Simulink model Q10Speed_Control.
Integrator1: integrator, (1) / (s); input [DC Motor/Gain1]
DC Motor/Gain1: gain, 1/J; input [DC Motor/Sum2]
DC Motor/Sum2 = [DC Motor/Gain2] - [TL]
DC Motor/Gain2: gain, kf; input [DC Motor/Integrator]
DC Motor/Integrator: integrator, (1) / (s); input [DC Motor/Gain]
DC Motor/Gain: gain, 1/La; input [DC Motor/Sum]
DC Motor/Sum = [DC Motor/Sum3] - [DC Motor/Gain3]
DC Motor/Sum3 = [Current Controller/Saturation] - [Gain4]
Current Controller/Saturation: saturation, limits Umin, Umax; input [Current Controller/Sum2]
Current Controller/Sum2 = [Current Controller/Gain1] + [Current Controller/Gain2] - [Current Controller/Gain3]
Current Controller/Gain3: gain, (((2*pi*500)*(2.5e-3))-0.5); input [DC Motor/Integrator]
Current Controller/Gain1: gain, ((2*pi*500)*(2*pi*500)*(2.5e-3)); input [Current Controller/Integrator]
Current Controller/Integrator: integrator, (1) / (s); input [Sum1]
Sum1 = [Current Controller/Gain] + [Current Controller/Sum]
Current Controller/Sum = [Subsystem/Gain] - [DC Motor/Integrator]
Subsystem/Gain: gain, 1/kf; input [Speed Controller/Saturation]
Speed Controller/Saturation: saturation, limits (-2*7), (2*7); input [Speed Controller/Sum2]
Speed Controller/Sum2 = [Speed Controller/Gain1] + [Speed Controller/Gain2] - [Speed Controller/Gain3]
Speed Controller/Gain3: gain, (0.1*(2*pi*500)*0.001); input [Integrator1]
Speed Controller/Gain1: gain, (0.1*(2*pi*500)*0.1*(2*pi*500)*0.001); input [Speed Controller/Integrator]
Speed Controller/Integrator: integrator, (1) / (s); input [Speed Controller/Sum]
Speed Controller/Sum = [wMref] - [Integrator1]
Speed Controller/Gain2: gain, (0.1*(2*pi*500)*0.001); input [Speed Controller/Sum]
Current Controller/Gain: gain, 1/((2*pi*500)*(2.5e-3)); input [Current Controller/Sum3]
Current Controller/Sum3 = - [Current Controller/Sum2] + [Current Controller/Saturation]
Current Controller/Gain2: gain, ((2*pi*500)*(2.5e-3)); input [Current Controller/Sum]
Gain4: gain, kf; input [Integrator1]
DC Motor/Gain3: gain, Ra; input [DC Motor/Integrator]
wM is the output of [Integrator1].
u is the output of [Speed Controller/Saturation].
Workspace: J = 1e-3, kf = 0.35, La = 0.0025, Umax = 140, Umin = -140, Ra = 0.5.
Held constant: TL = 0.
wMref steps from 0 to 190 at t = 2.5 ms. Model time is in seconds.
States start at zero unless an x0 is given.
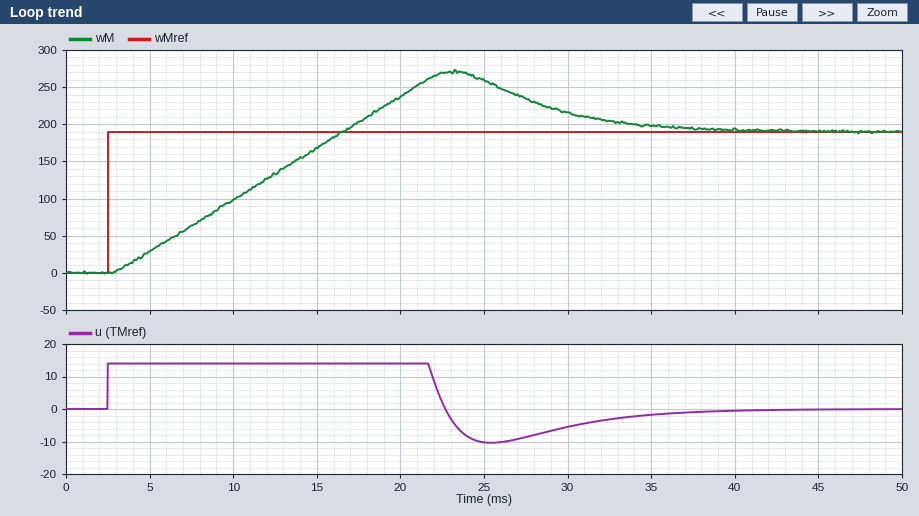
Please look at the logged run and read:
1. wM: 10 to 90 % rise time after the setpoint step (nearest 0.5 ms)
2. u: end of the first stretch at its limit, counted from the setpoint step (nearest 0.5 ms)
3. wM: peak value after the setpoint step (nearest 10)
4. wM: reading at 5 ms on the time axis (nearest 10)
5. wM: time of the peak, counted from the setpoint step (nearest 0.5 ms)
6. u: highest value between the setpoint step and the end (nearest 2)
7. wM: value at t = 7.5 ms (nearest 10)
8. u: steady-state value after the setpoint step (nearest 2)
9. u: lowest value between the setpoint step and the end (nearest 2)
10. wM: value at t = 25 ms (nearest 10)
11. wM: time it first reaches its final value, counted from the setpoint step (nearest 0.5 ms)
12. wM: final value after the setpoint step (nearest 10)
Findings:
11.0 ms
19.0 ms
270
30
20.5 ms
14
60
0
-10
260
14.0 ms
190
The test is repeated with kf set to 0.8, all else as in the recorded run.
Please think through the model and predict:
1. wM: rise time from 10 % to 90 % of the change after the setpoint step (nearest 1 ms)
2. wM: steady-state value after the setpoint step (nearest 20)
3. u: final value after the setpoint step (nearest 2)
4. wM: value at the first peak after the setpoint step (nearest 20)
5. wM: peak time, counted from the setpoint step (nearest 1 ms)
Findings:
10 ms
180
14
200
16 ms
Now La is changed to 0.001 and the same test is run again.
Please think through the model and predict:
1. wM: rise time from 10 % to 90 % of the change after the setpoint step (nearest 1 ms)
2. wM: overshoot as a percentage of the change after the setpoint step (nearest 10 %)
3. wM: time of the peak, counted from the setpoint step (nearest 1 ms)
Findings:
11 ms
40 %
20 ms
